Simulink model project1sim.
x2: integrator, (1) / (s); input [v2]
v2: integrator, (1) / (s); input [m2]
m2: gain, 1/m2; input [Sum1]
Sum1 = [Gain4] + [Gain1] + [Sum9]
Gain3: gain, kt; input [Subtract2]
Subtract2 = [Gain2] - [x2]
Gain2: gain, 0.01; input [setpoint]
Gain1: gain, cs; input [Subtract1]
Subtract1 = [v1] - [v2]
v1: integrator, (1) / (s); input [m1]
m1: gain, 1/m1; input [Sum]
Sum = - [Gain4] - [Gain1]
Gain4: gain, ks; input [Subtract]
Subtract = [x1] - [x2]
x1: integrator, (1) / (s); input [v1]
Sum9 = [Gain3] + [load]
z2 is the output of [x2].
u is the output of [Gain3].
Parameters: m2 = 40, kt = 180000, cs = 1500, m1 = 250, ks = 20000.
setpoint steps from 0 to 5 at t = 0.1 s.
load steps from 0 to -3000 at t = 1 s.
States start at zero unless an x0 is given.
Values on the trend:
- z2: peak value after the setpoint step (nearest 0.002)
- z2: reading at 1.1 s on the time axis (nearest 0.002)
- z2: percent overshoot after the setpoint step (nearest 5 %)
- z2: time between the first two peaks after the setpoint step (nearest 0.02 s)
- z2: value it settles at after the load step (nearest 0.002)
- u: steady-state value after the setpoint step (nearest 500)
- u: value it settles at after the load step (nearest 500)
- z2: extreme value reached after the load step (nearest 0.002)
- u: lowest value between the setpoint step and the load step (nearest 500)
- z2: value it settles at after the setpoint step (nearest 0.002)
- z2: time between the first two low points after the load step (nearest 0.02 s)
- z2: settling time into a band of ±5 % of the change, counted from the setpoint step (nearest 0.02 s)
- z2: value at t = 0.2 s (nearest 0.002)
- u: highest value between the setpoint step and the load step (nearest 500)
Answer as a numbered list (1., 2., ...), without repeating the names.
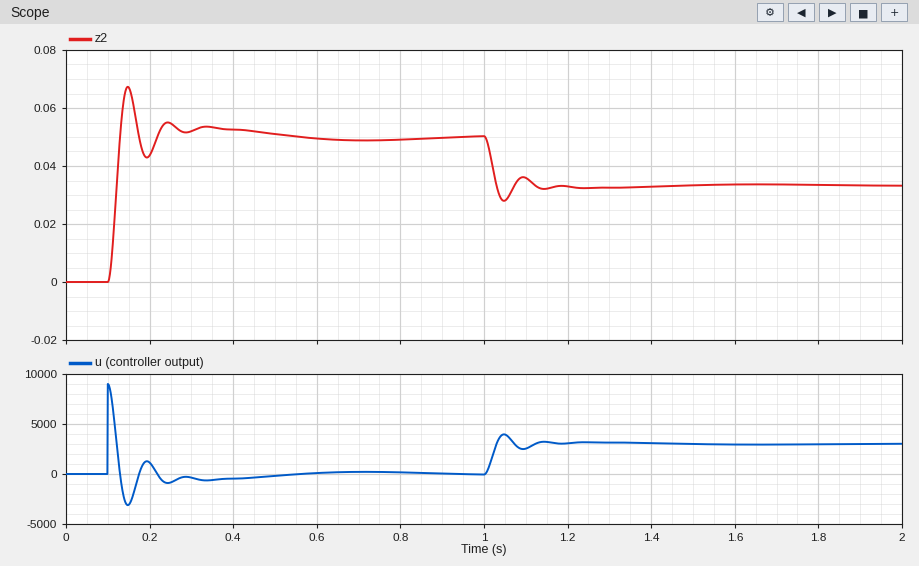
1. 0.068
2. 0.036
3. 35 %
4. 0.10 s
5. 0.034
6. 0
7. 3000
8. 0.028
9. -3000
10. 0.050
11. 0.10 s
12. 0.32 s
13. 0.044
14. 9000
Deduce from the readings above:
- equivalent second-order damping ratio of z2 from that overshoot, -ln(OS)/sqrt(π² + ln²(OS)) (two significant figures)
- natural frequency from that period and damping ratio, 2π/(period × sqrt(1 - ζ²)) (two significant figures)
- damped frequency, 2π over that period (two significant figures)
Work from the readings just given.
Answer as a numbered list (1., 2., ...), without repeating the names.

1. 0.32
2. 66 rad/s
3. 63 rad/s
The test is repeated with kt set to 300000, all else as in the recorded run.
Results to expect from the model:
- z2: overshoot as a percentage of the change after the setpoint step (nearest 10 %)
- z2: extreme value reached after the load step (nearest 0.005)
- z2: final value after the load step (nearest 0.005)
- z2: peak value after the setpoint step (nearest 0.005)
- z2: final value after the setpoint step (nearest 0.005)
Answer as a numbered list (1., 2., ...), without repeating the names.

1. 50 %
2. 0.035
3. 0.040
4. 0.075
5. 0.050
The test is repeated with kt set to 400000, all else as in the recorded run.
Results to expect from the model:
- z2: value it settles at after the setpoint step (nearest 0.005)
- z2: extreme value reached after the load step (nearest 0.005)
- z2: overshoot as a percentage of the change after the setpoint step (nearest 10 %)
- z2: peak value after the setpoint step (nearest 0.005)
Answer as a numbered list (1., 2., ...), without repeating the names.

1. 0.050
2. 0.040
3. 50 %
4. 0.075
